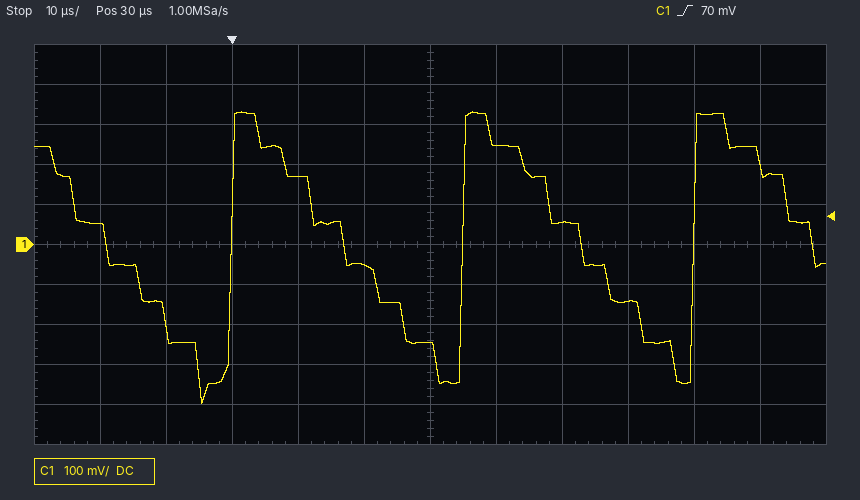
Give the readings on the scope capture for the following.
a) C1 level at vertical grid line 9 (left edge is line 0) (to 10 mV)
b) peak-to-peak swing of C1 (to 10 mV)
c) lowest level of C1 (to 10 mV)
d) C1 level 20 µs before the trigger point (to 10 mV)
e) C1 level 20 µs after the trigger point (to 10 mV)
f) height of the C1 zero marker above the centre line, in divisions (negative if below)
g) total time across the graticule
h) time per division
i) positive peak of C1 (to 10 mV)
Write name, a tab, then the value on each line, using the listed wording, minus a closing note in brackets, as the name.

C1 level at vertical grid line 9 (left edge is line 0)	-140 mV
peak-to-peak swing of C1	730 mV
lowest level of C1	-400 mV
C1 level 20 µs before the trigger point	50 mV
C1 level 20 µs after the trigger point	-50 mV
height of the C1 zero marker above the centre line, in divisions	0.0 div
total time across the graticule	120 µs
time per division	10 µs
positive peak of C1	330 mV
